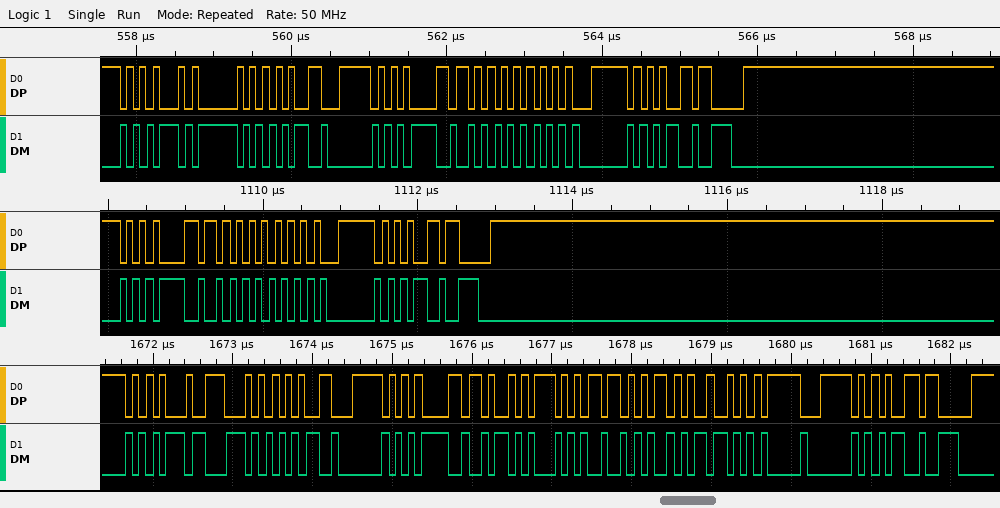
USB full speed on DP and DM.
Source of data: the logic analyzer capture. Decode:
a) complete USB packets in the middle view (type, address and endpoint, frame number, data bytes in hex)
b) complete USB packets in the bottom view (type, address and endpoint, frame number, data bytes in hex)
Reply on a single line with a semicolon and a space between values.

DATA1 [ ], ACK; IN ADDR 3 EP 0, DATA1 [ 04 03 09 04 ], ACK
